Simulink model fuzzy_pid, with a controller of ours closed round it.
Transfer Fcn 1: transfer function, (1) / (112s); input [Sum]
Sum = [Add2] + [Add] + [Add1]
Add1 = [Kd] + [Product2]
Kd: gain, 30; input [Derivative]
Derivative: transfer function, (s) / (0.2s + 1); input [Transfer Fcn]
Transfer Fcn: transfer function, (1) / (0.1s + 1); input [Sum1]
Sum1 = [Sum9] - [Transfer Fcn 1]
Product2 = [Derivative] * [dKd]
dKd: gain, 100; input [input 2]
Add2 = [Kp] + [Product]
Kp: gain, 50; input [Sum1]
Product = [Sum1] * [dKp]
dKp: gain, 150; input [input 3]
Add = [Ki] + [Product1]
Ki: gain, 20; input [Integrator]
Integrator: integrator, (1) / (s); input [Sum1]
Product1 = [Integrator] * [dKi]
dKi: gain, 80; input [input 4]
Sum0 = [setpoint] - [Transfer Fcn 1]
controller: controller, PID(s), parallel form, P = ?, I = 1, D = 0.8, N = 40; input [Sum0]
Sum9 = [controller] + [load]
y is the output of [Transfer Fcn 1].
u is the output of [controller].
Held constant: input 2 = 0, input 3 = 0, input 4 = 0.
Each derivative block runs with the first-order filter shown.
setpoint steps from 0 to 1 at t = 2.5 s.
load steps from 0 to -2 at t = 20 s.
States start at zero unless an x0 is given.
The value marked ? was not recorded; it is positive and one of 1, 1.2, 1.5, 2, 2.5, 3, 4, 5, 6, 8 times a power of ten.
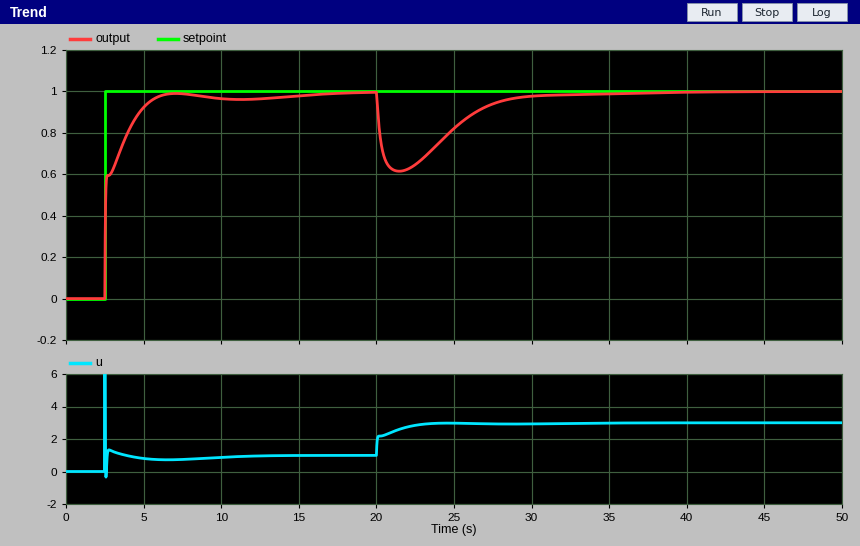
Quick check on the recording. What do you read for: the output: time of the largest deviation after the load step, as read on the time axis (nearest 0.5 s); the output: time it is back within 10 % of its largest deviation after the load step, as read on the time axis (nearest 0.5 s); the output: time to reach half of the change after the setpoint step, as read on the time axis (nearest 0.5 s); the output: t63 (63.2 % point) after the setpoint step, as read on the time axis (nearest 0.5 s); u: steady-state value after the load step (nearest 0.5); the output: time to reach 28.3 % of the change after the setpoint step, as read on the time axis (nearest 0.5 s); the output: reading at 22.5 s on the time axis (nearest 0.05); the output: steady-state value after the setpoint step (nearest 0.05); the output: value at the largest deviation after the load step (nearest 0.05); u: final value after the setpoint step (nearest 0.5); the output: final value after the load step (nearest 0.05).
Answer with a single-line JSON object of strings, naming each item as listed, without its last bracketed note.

{"the output: time of the largest deviation after the load step, as read on the time axis": "21.5 s", "the output: time it is back within 10 % of its largest deviation after the load step, as read on the time axis": "28.5 s", "the output: time to reach half of the change after the setpoint step, as read on the time axis": "2.5 s", "the output: t63 (63.2 % point) after the setpoint step, as read on the time axis": "3.0 s", "u: steady-state value after the load step": "3.0", "the output: time to reach 28.3 % of the change after the setpoint step, as read on the time axis": "2.5 s", "the output: reading at 22.5 s on the time axis": "0.65", "the output: steady-state value after the setpoint step": "1.00", "the output: value at the largest deviation after the load step": "0.60", "u: final value after the setpoint step": "1.0", "the output: final value after the load step": "1.00"}
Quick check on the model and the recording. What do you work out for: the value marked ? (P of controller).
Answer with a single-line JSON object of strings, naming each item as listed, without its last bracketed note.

{"the value marked ?": "3"}
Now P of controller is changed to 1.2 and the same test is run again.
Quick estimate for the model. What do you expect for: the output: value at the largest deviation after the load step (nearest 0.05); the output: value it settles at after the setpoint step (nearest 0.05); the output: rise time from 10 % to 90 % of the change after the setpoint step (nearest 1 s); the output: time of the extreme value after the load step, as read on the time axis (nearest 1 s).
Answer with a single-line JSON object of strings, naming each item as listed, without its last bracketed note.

{"the output: value at the largest deviation after the load step": "0.45", "the output: value it settles at after the setpoint step": "1.00", "the output: rise time from 10 % to 90 % of the change after the setpoint step": "3 s", "the output: time of the extreme value after the load step, as read on the time axis": "22 s"}
